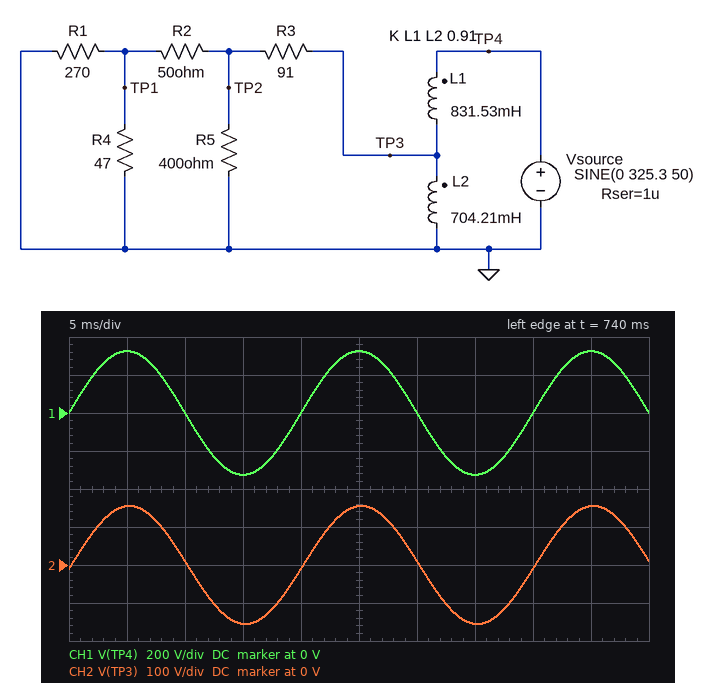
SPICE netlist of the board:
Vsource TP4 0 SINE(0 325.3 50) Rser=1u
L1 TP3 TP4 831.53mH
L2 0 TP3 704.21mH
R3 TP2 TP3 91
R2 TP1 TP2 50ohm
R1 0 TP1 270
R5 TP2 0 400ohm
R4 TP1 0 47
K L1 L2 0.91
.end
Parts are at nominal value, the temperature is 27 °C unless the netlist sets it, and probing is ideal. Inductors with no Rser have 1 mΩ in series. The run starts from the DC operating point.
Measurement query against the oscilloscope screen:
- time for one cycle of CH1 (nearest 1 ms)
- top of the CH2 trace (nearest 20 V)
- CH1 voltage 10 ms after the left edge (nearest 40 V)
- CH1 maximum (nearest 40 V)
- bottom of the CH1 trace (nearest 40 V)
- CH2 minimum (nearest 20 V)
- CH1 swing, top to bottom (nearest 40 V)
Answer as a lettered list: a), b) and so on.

a) 20 ms
b) 160 V
c) 0 V
d) 320 V
e) -320 V
f) -160 V
g) 640 V
